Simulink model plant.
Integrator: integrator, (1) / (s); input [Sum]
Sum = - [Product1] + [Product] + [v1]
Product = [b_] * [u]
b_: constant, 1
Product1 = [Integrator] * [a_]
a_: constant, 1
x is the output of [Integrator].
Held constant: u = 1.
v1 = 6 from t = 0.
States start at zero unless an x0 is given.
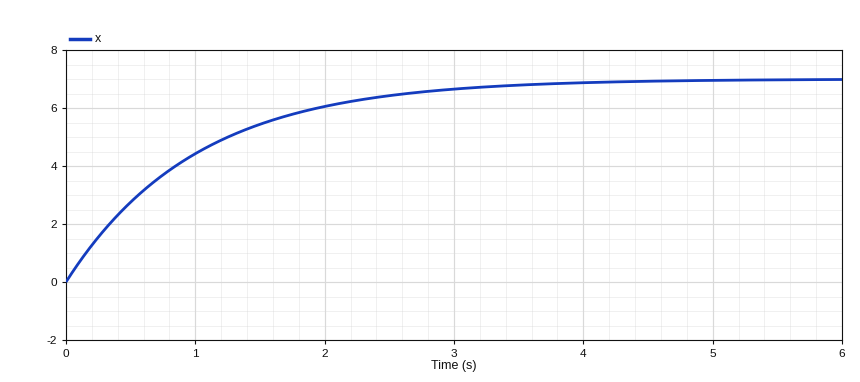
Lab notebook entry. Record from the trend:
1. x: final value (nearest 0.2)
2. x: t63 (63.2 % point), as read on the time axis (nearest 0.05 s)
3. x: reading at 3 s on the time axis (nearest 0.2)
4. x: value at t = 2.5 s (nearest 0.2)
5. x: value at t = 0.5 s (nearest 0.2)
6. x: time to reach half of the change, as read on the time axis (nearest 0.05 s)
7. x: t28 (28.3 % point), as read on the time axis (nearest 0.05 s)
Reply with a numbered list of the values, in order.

1. 7.0
2. 1.00 s
3. 6.6
4. 6.4
5. 2.8
6. 0.70 s
7. 0.35 s
